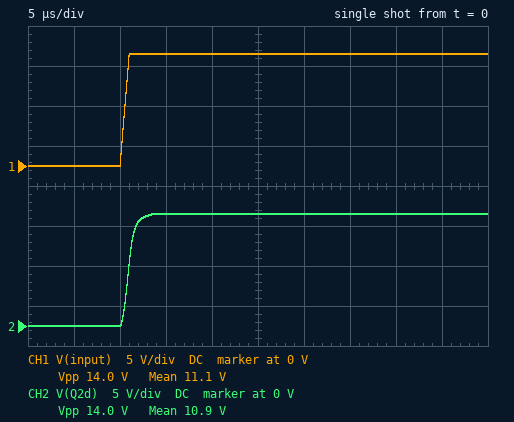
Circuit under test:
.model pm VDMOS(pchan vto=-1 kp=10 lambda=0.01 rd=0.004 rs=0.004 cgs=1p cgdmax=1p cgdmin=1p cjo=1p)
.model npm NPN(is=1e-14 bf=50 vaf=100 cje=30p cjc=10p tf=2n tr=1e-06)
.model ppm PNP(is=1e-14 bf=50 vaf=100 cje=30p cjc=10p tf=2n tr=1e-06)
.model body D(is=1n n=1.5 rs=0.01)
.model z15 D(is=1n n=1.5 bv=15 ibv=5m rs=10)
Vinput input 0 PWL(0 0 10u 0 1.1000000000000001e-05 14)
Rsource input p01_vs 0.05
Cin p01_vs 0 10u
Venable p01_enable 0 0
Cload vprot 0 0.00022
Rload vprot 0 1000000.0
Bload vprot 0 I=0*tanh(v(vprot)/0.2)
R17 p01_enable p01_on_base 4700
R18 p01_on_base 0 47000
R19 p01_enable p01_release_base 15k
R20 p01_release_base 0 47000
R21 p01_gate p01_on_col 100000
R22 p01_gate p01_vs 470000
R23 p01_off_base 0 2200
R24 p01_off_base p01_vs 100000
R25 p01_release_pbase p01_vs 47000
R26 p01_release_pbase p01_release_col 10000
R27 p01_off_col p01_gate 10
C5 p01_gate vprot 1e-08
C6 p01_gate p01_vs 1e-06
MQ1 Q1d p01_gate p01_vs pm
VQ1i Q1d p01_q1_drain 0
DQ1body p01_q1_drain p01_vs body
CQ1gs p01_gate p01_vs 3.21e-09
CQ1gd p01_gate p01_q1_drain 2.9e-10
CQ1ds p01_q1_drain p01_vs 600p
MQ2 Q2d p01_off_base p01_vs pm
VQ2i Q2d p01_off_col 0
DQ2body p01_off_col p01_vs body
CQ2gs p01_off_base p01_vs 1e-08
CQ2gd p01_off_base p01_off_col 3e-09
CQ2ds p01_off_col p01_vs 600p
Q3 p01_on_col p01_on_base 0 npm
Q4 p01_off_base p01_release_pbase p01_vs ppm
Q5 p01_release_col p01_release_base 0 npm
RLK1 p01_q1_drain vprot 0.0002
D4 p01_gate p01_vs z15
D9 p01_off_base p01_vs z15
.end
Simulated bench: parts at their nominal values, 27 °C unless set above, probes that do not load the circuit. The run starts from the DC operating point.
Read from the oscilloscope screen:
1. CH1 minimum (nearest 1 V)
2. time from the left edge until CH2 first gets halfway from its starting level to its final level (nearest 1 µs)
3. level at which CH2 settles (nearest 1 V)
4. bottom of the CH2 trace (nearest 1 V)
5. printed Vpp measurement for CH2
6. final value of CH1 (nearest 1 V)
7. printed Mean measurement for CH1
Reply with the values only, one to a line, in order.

0 V
11 µs
14 V
0 V
14.0 V
14 V
11.1 V
